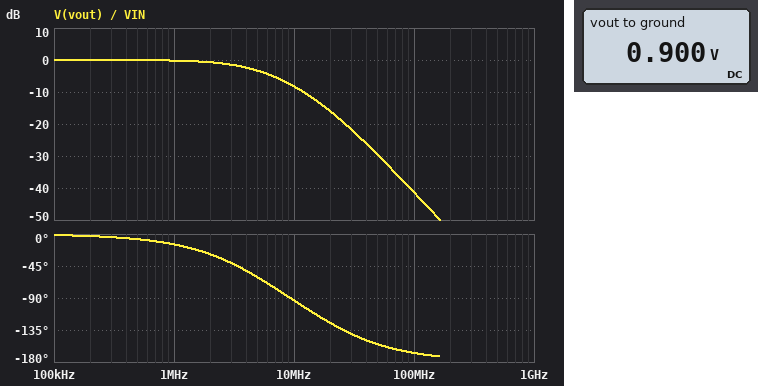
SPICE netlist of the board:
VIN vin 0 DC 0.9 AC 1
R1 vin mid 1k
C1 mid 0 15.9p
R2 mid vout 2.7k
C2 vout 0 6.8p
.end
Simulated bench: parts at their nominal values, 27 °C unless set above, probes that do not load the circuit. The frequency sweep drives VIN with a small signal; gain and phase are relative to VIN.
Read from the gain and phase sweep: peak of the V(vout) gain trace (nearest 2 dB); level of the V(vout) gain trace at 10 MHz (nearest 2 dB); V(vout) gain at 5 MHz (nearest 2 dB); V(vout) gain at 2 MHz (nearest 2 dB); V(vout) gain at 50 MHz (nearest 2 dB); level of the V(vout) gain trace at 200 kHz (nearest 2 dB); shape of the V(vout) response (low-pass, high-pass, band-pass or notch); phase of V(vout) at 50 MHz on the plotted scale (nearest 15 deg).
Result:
0 dB
-8 dB
-4 dB
0 dB
-30 dB
0 dB
low-pass
-150 deg
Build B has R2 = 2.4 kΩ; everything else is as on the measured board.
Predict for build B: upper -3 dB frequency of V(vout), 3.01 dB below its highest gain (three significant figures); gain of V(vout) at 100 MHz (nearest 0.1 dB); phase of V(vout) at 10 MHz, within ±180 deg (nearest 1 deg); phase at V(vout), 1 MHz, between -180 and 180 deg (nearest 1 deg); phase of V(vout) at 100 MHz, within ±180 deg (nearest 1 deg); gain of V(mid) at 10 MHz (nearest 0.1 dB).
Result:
4.87 MHz
-40.4 dB
-91 deg
-14 deg
-166 deg
-4.7 dB
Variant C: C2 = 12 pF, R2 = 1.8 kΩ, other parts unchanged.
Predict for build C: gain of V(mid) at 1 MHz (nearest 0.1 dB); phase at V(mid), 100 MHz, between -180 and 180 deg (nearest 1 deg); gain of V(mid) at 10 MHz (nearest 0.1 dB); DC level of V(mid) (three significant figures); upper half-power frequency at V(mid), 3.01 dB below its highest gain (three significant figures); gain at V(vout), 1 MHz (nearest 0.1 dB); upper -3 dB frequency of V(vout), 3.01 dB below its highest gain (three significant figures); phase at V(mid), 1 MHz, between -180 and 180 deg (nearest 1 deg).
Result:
-0.2 dB
-81 deg
-5.4 dB
900 mV
5.15 MHz
-0.3 dB
3.72 MHz
-10 deg
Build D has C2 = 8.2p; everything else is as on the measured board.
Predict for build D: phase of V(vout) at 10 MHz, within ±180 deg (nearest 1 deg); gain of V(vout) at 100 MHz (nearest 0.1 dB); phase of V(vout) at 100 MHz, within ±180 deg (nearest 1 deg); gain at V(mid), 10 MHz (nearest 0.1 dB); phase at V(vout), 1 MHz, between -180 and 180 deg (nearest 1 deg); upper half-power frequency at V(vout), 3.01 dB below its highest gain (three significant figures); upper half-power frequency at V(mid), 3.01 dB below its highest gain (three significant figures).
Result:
-98 deg
-43.0 dB
-168 deg
-4.7 dB
-16 deg
4.09 MHz
6.26 MHz
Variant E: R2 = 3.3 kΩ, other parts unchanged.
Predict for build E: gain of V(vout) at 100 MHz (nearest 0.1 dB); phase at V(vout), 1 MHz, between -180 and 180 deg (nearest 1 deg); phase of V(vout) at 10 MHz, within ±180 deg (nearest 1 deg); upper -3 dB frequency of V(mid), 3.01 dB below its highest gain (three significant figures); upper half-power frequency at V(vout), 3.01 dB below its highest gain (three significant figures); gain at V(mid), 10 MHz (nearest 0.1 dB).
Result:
-43.1 dB
-16 deg
-98 deg
6.79 MHz
4.23 MHz
-4.4 dB
